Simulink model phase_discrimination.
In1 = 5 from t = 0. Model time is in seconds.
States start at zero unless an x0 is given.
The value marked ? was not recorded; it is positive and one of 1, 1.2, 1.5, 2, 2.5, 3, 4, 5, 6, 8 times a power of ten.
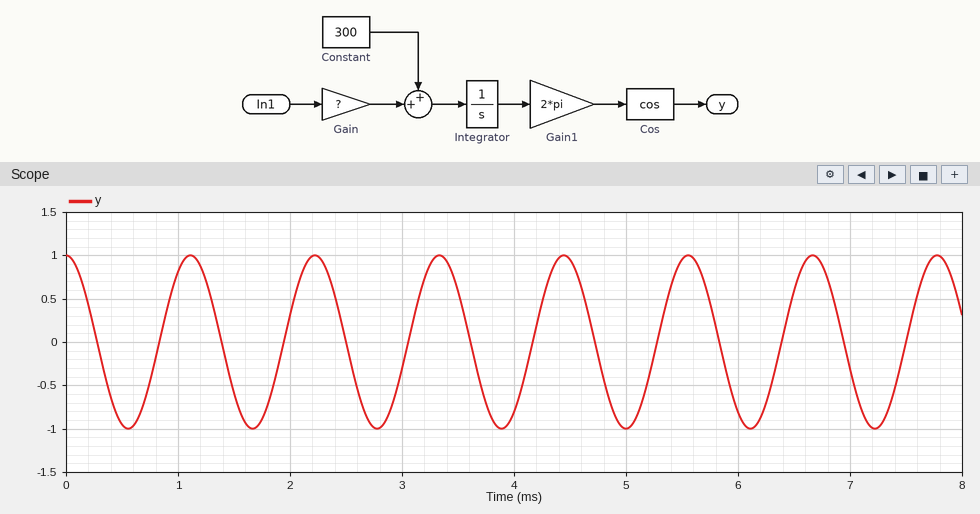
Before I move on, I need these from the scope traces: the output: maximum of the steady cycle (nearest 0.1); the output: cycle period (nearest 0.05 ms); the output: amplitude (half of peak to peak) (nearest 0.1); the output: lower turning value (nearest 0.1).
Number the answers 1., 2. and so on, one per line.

1. 1.0
2. 1.10 ms
3. 1.0
4. -1.0
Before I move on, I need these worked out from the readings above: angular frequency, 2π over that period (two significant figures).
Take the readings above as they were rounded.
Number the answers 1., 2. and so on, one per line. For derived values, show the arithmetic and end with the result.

1. 2π / 1.1 = 5.7 rad/ms
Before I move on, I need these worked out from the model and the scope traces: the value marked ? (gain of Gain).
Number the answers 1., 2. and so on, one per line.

1. 120
